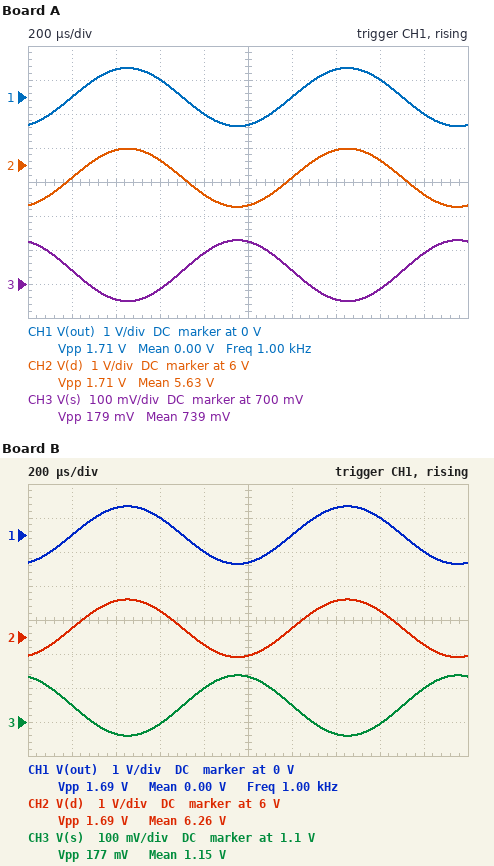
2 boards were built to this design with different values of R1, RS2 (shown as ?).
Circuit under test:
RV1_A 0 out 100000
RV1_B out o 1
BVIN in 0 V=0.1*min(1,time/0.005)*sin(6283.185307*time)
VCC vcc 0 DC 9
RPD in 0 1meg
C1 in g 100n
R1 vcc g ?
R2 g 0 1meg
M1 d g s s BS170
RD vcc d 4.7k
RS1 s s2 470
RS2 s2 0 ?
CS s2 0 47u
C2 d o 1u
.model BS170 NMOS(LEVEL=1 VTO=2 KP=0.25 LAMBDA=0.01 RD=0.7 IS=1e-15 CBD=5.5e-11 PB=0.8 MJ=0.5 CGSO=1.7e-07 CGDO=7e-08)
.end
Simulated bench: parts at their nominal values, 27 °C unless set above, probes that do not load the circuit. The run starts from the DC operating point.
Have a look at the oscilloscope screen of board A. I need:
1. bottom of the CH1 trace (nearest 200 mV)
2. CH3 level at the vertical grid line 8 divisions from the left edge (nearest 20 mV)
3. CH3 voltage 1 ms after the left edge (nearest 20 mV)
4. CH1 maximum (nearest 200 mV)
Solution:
-800 mV
680 mV
820 mV
800 mV
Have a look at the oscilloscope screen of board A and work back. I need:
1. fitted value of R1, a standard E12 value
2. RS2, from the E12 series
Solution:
2.2 MΩ
560 Ω
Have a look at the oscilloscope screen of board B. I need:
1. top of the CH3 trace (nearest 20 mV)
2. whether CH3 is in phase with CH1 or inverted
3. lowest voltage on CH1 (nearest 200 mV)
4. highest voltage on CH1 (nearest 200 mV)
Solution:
1.24 V
inverted
-800 mV
800 mV
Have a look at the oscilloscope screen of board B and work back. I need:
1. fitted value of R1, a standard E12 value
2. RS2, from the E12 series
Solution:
1.8 MΩ
1.5 kΩ
